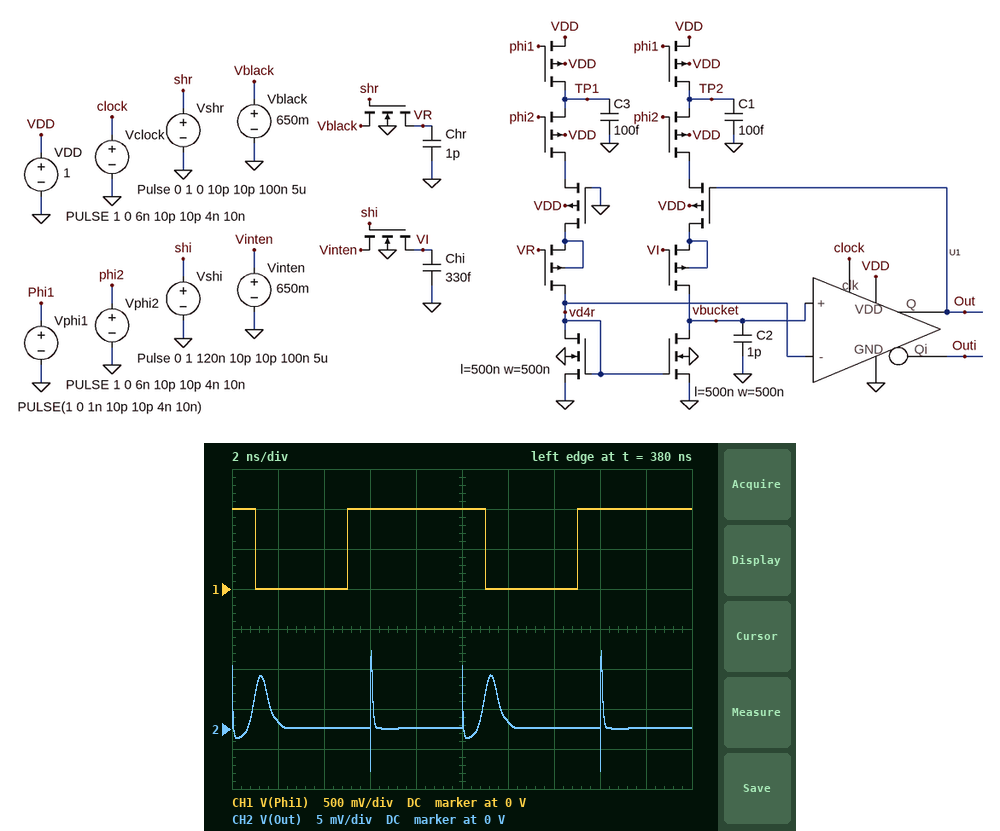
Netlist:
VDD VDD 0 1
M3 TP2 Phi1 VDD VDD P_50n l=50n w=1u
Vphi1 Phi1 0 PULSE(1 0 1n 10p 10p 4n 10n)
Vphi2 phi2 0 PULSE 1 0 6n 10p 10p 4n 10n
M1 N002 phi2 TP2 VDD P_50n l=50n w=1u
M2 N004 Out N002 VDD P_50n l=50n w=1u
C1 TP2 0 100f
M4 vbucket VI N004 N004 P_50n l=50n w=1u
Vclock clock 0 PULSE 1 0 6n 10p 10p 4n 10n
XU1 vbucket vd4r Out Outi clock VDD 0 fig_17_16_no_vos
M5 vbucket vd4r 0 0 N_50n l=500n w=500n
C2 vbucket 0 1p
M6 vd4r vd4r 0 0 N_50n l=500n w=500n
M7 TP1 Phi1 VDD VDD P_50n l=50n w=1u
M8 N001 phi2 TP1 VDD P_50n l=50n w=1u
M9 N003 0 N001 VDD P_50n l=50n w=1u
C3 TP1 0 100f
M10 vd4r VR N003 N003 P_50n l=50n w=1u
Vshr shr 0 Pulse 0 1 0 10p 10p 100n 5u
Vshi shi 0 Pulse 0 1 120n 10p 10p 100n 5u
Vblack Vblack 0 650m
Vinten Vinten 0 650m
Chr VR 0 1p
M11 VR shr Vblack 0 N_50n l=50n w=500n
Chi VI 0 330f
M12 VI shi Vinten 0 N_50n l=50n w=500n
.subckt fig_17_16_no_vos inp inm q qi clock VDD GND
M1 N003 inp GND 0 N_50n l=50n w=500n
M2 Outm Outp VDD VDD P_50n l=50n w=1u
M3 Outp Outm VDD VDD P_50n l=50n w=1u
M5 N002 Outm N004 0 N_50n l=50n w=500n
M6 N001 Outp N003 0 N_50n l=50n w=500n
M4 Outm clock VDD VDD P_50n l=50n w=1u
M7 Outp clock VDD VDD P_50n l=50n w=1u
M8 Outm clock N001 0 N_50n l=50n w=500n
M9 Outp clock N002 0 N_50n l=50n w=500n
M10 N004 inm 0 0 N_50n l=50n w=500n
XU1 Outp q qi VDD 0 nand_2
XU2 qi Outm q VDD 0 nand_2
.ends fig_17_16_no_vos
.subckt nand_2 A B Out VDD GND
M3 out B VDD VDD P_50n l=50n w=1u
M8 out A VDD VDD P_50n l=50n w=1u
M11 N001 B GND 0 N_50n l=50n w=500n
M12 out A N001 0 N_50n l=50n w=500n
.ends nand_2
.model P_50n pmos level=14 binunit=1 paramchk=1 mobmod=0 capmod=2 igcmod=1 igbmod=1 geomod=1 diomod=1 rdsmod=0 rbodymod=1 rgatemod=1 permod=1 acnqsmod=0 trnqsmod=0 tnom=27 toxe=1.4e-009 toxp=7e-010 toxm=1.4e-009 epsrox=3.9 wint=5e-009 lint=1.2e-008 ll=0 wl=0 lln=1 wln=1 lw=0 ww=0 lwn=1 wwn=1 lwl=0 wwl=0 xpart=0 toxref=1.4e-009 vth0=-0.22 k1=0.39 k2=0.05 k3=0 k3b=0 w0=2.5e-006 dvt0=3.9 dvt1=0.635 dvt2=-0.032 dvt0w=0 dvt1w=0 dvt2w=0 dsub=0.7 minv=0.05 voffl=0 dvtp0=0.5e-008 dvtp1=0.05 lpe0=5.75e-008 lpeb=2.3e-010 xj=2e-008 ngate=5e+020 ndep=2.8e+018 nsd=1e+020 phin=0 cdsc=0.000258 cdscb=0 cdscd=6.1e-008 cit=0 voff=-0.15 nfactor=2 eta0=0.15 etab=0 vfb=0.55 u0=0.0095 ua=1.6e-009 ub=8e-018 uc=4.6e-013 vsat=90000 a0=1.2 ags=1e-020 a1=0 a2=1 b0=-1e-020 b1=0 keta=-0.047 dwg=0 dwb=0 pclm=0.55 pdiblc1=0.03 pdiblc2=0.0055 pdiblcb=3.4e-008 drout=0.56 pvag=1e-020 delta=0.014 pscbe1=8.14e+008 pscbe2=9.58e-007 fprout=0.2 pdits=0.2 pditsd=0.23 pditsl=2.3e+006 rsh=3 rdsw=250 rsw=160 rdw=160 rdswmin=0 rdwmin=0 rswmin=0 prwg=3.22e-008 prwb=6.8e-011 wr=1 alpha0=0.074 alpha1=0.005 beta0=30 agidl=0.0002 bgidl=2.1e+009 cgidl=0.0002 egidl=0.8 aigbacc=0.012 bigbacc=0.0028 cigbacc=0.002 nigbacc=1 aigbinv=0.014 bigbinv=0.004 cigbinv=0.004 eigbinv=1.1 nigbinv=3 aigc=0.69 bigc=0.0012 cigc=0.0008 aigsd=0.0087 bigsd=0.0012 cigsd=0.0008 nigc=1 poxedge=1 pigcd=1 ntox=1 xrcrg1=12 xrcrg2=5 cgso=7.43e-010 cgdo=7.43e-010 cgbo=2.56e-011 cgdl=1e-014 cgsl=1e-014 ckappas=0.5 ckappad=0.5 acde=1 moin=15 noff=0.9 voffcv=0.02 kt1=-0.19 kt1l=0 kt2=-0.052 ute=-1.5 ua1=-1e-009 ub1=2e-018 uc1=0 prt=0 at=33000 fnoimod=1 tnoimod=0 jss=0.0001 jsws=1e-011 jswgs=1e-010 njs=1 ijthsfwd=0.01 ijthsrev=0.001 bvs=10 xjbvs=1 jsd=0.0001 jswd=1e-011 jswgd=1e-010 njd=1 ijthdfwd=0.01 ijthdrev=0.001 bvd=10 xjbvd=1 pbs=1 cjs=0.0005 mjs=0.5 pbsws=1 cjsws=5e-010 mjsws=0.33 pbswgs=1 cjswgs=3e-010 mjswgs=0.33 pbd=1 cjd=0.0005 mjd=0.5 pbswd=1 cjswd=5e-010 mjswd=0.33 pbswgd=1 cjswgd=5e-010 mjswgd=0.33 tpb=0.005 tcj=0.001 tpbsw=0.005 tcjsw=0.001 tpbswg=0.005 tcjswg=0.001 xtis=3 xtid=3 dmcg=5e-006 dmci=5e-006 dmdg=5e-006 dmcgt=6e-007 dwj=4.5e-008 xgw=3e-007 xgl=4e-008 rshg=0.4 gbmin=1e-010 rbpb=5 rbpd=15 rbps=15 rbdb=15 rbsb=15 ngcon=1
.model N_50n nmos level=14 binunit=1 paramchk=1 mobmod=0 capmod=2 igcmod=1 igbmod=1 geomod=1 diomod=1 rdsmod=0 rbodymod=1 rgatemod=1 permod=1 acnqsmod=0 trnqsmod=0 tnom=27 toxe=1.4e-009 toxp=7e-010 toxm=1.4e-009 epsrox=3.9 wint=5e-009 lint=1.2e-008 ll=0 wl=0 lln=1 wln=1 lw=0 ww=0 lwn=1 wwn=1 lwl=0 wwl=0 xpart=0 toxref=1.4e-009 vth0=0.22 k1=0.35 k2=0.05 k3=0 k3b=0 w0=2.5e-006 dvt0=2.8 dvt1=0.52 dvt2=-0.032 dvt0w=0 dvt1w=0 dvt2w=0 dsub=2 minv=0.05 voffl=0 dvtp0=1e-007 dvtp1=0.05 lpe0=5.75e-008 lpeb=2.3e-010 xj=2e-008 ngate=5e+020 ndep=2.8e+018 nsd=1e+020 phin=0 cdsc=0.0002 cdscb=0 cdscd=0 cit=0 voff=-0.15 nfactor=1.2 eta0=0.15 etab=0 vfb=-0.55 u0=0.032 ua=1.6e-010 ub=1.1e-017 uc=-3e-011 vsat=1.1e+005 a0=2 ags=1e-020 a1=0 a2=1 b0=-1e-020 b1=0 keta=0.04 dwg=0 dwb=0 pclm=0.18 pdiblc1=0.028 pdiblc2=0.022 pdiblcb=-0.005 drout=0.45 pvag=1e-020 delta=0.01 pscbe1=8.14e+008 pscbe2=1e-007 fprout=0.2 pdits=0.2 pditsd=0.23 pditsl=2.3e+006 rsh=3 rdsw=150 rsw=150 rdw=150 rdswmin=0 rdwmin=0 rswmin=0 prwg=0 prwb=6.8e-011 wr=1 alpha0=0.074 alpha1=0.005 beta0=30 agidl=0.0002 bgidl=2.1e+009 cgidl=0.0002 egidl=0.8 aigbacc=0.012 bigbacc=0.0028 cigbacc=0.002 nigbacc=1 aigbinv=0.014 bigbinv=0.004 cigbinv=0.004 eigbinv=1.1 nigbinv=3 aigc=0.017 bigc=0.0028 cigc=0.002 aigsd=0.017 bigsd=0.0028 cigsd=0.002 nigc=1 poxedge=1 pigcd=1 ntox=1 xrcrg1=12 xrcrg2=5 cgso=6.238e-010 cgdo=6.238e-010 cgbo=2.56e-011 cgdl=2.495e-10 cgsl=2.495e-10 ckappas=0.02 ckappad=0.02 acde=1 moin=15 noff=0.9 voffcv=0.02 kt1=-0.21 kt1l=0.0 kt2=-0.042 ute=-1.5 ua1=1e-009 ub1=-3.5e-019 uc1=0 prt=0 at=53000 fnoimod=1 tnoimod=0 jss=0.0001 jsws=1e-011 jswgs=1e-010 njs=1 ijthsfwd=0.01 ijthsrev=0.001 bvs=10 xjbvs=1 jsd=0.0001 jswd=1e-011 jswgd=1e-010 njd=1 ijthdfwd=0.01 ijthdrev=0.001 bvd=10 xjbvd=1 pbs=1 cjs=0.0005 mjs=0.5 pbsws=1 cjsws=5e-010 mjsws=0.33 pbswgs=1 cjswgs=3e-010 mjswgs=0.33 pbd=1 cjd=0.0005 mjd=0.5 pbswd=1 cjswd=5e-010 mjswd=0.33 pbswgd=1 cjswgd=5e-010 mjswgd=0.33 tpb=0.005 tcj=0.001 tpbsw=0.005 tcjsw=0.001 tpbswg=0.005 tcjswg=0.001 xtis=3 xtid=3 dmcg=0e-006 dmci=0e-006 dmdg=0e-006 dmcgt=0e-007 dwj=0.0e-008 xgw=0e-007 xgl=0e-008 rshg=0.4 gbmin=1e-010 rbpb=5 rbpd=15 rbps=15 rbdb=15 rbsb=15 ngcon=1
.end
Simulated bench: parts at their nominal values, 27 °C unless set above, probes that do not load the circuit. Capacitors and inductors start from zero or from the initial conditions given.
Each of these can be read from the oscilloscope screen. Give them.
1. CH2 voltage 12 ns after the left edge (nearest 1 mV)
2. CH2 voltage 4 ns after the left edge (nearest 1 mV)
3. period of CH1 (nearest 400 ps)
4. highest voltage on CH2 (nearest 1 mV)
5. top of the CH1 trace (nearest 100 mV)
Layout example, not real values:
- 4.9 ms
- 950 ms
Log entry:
- 1 mV
- 0 V
- 10.0 ns
- 10 mV
- 1.0 V
